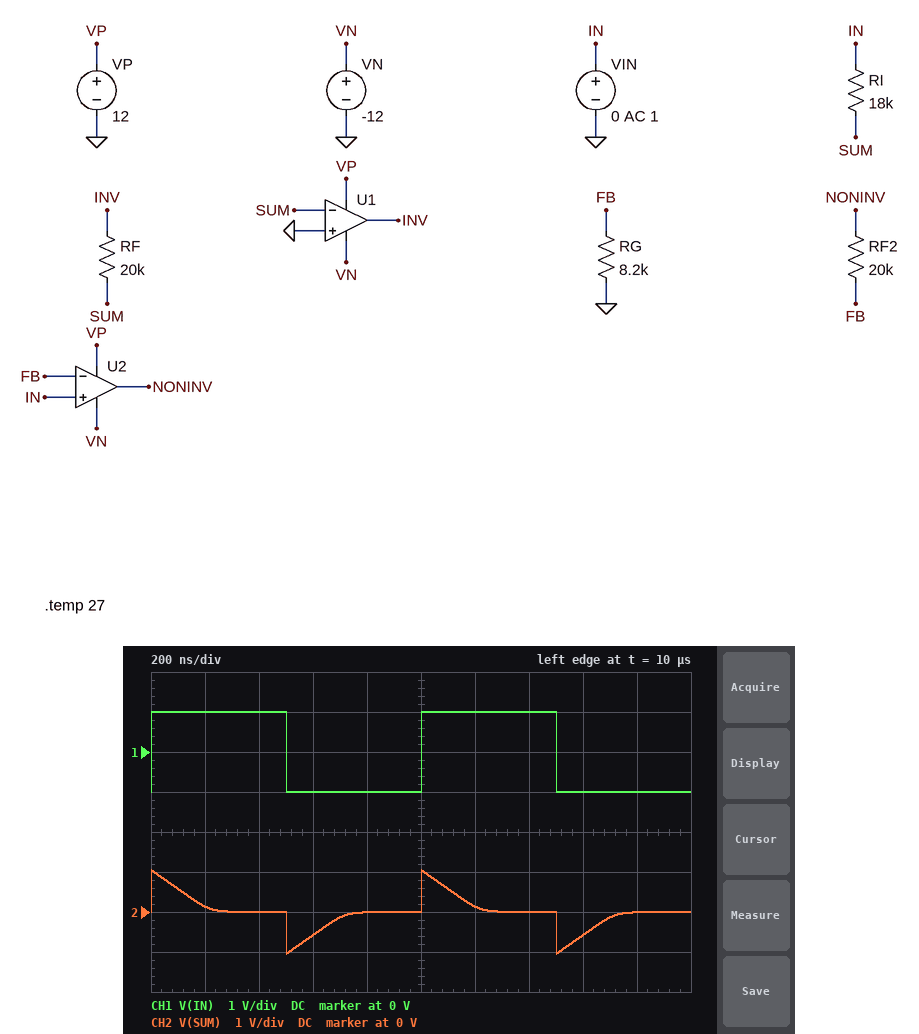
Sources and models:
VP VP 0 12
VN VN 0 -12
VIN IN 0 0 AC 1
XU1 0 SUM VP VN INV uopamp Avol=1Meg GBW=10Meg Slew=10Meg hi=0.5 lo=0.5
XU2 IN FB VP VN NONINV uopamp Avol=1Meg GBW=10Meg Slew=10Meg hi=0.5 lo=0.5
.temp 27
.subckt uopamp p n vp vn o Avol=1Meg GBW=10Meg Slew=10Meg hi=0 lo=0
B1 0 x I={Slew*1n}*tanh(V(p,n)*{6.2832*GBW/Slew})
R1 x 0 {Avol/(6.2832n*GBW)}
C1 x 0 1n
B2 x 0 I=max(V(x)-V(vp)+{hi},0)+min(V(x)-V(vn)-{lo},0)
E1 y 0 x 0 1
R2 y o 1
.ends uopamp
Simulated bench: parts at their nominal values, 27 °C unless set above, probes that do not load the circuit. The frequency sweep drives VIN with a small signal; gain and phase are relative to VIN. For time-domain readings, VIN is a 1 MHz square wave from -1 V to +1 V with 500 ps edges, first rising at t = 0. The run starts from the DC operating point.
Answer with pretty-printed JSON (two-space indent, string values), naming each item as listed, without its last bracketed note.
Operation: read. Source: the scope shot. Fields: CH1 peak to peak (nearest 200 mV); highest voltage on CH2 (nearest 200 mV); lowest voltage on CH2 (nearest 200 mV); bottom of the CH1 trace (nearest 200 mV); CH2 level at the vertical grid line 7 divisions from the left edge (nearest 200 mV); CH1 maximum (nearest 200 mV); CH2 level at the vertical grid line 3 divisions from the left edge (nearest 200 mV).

{
  "CH1 peak to peak": "2.0 V",
  "highest voltage on CH2": "1.0 V",
  "lowest voltage on CH2": "-1.0 V",
  "bottom of the CH1 trace": "-1.0 V",
  "CH2 level at the vertical grid line 7 divisions from the left edge": "0 V",
  "CH1 maximum": "1.0 V",
  "CH2 level at the vertical grid line 3 divisions from the left edge": "-600 mV"
}
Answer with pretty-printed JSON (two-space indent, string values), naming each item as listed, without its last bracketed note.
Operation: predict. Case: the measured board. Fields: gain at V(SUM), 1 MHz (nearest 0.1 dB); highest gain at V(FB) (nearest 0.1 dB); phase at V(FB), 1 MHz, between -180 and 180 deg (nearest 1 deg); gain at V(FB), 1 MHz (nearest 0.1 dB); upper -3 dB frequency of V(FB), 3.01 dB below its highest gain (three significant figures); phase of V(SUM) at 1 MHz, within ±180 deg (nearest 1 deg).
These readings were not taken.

{
  "gain at V(SUM), 1 MHz": "-19.3 dB",
  "highest gain at V(FB)": "0 dB",
  "phase at V(FB), 1 MHz, between -180 and 180 deg": "-19 deg",
  "gain at V(FB), 1 MHz": "-0.5 dB",
  "upper -3 dB frequency of V(FB), 3.01 dB below its highest gain": "2.91 MHz",
  "phase of V(SUM) at 1 MHz, within ±180 deg": "78 deg"
}
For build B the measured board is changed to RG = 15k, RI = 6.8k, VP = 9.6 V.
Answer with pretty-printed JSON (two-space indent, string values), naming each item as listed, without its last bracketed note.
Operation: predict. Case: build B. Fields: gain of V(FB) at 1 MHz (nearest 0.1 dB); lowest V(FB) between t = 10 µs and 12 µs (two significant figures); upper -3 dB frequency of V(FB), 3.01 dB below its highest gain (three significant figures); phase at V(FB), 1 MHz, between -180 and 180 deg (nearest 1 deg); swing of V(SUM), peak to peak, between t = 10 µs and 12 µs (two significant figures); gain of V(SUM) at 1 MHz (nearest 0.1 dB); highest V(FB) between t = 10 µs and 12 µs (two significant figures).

{
  "gain of V(FB) at 1 MHz": "-0.2 dB",
  "lowest V(FB) between t = 10 µs and 12 µs": "-970 mV",
  "upper -3 dB frequency of V(FB), 3.01 dB below its highest gain": "4.29 MHz",
  "phase at V(FB), 1 MHz, between -180 and 180 deg": "-13 deg",
  "swing of V(SUM), peak to peak, between t = 10 µs and 12 µs": "2.7 V",
  "gain of V(SUM) at 1 MHz": "-11.3 dB",
  "highest V(FB) between t = 10 µs and 12 µs": "970 mV"
}
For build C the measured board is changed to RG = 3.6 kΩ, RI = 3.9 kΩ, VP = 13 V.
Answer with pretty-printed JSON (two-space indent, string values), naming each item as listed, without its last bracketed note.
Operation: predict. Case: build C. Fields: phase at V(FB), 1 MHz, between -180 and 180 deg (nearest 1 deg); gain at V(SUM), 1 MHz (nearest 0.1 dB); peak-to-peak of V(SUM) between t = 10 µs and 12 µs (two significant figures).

{
  "phase at V(FB), 1 MHz, between -180 and 180 deg": "-33 deg",
  "gain at V(SUM), 1 MHz": "-7.2 dB",
  "peak-to-peak of V(SUM) between t = 10 µs and 12 µs": "2.5 V"
}
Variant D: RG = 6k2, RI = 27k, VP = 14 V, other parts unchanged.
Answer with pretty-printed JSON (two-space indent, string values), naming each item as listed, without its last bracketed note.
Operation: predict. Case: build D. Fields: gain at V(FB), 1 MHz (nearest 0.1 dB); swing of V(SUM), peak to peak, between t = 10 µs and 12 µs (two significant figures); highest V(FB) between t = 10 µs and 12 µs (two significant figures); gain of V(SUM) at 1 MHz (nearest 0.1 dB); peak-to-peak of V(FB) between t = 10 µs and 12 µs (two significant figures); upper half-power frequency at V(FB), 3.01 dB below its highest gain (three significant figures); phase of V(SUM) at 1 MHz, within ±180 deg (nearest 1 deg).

{
  "gain at V(FB), 1 MHz": "-0.7 dB",
  "swing of V(SUM), peak to peak, between t = 10 µs and 12 µs": "1.7 V",
  "highest V(FB) between t = 10 µs and 12 µs": "430 mV",
  "gain of V(SUM) at 1 MHz": "-22.7 dB",
  "peak-to-peak of V(FB) between t = 10 µs and 12 µs": "1.2 V",
  "upper half-power frequency at V(FB), 3.01 dB below its highest gain": "2.37 MHz",
  "phase of V(SUM) at 1 MHz, within ±180 deg": "80 deg"
}
